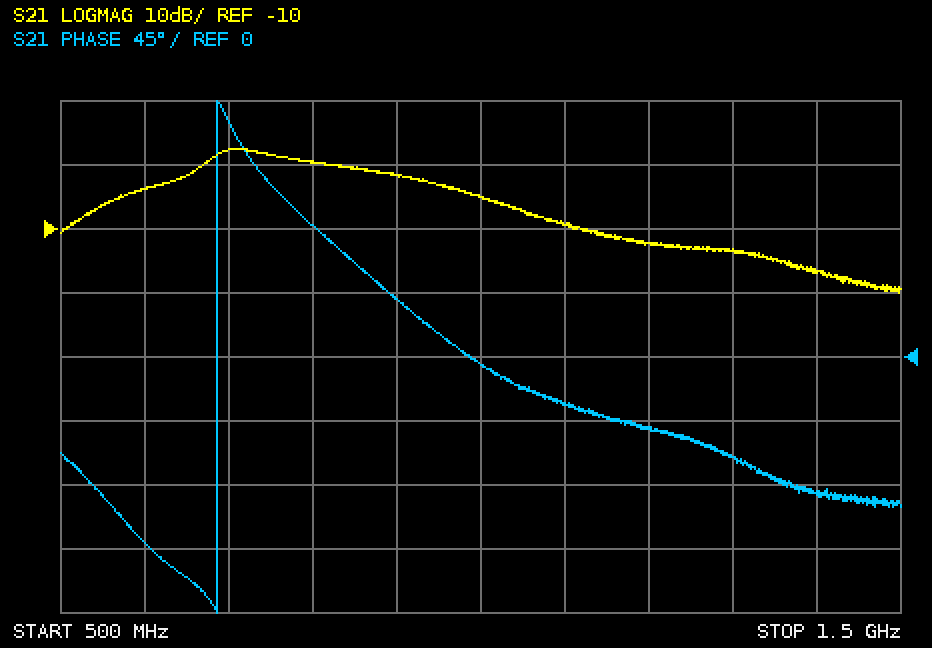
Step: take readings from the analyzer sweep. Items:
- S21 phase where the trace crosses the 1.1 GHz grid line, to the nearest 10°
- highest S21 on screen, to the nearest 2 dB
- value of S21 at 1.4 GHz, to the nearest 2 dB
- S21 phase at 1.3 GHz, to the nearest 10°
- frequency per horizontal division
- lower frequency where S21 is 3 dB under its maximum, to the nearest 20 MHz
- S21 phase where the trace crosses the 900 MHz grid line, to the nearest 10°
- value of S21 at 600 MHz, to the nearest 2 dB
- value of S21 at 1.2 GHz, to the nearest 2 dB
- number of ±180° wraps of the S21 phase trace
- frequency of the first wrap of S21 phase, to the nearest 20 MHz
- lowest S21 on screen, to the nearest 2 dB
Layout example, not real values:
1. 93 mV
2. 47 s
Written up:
1. -30°
2. 2 dB
3. -16 dB
4. -70°
5. 100 MHz
6. 660 MHz
7. 40°
8. -4 dB
9. -12 dB
10. 1
11. 680 MHz
12. -20 dB
